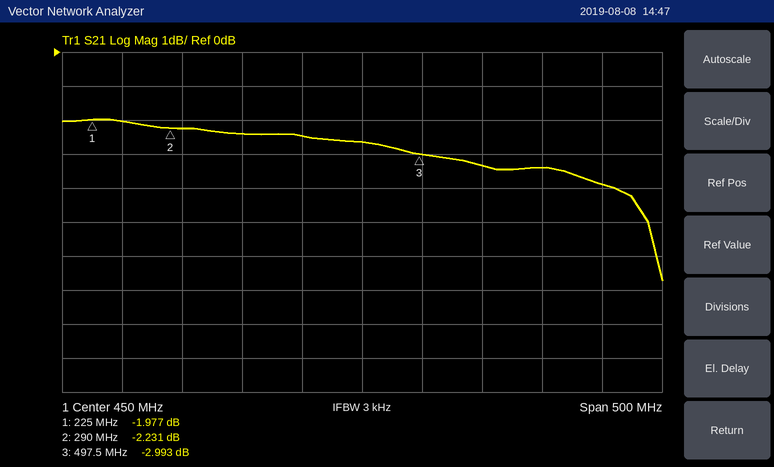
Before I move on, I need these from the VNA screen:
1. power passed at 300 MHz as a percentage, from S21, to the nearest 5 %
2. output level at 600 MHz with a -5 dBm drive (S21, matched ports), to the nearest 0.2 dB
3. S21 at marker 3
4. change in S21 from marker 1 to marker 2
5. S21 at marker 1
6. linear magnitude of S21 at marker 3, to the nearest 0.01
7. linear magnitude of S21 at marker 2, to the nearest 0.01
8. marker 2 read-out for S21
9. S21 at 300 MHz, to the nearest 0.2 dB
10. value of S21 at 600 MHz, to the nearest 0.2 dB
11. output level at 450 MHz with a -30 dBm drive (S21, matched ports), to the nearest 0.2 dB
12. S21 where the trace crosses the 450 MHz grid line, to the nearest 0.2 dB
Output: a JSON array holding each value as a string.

["60 %", "-8.4 dBm", "-2.993 dB", "-0.254 dB", "-1.977 dB", "0.71", "0.77", "-2.231 dB", "-2.2 dB", "-3.4 dB", "-32.6 dBm", "-2.6 dB"]
